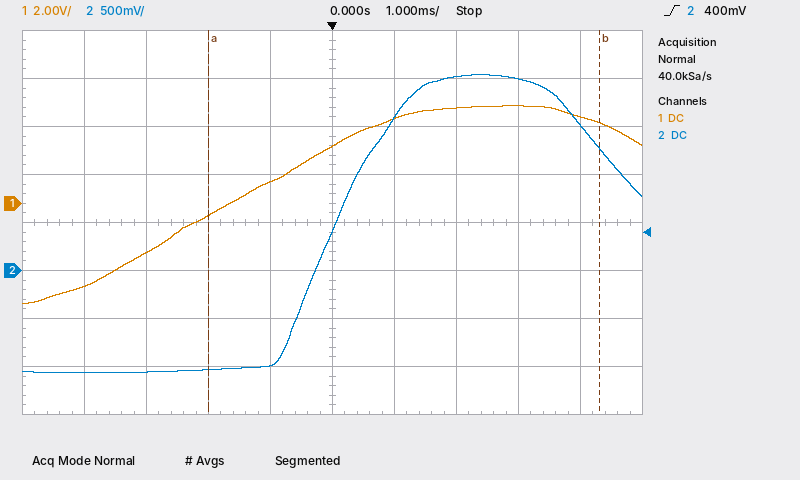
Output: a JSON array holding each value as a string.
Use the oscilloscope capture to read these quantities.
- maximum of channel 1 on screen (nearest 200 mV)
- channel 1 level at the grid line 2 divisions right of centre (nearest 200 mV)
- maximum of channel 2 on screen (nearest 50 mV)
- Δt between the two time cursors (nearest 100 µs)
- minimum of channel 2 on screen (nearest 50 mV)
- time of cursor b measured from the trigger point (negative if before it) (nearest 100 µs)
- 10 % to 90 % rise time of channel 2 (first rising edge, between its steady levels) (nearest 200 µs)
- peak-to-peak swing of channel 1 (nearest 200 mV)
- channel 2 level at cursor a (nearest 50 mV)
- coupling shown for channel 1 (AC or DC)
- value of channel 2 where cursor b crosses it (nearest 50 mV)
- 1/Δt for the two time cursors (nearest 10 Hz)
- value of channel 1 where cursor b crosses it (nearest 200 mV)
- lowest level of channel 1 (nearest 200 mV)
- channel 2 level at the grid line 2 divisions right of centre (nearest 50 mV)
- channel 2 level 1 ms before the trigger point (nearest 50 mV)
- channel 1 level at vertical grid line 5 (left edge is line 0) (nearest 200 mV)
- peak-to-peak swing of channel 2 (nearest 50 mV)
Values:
["4.0 V", "4.0 V", "2.05 V", "6.3 ms", "-1.05 V", "+4.3 ms", "1.8 ms", "8.2 V", "-1.05 V", "DC", "1.25 V", "160 Hz", "3.4 V", "-4.2 V", "2.00 V", "-1.00 V", "2.4 V", "3.10 V"]
